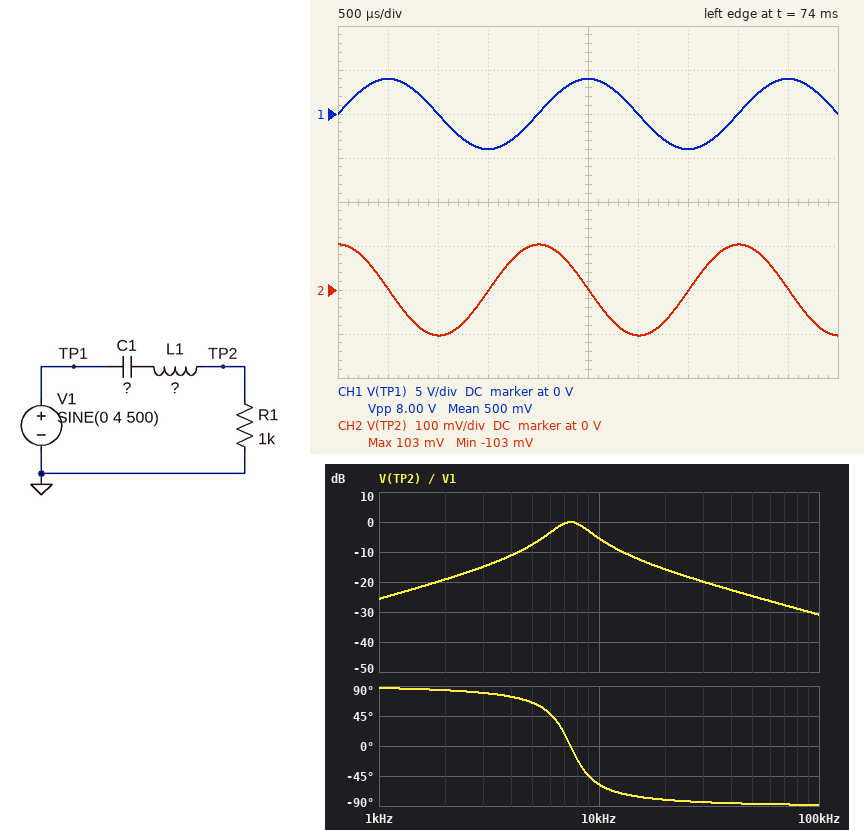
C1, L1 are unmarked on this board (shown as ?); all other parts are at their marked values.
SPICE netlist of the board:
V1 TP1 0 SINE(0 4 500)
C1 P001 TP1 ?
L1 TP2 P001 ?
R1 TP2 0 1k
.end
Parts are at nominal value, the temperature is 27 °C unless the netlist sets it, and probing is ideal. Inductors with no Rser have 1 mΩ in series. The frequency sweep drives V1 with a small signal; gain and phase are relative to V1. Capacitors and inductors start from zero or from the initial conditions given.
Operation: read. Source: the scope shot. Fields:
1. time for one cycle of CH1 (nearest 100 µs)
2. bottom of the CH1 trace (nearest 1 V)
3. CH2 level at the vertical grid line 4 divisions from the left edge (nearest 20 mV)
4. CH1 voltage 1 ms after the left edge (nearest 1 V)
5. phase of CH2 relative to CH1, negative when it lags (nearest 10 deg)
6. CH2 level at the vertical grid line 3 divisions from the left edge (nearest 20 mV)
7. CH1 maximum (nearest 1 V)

2.0 ms
-4 V
100 mV
0 V
90 deg
0 V
4 V
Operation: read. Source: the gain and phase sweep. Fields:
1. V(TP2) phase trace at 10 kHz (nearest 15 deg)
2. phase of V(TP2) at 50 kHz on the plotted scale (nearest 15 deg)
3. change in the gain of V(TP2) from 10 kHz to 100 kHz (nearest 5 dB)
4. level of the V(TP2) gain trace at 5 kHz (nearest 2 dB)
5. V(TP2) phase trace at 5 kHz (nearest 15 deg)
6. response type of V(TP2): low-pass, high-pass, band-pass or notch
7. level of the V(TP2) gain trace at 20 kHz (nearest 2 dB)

-60 deg
-90 deg
-25 dB
-8 dB
60 deg
band-pass
-16 dB
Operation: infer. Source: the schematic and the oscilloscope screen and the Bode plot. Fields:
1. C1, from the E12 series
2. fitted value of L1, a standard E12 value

8.2 nF
56 mH
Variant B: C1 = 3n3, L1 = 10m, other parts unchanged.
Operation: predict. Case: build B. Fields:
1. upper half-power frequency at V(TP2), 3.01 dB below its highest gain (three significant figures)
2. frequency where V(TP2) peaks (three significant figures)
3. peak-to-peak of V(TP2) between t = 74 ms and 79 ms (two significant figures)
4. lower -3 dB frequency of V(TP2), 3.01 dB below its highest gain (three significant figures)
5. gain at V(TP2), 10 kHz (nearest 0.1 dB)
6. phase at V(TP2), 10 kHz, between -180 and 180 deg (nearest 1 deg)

36.8 kHz
27.7 kHz
83 mV
20.9 kHz
-12.7 dB
77 deg
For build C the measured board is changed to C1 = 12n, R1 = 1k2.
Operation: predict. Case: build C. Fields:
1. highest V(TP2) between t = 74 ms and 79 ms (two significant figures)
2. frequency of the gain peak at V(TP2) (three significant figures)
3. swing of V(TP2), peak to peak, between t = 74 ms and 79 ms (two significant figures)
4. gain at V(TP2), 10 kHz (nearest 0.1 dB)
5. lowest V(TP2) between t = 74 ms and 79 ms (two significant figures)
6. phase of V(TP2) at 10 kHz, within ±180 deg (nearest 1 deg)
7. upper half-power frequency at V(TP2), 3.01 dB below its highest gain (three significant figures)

180 mV
6.14 kHz
360 mV
-6.4 dB
-180 mV
-61 deg
8.08 kHz
